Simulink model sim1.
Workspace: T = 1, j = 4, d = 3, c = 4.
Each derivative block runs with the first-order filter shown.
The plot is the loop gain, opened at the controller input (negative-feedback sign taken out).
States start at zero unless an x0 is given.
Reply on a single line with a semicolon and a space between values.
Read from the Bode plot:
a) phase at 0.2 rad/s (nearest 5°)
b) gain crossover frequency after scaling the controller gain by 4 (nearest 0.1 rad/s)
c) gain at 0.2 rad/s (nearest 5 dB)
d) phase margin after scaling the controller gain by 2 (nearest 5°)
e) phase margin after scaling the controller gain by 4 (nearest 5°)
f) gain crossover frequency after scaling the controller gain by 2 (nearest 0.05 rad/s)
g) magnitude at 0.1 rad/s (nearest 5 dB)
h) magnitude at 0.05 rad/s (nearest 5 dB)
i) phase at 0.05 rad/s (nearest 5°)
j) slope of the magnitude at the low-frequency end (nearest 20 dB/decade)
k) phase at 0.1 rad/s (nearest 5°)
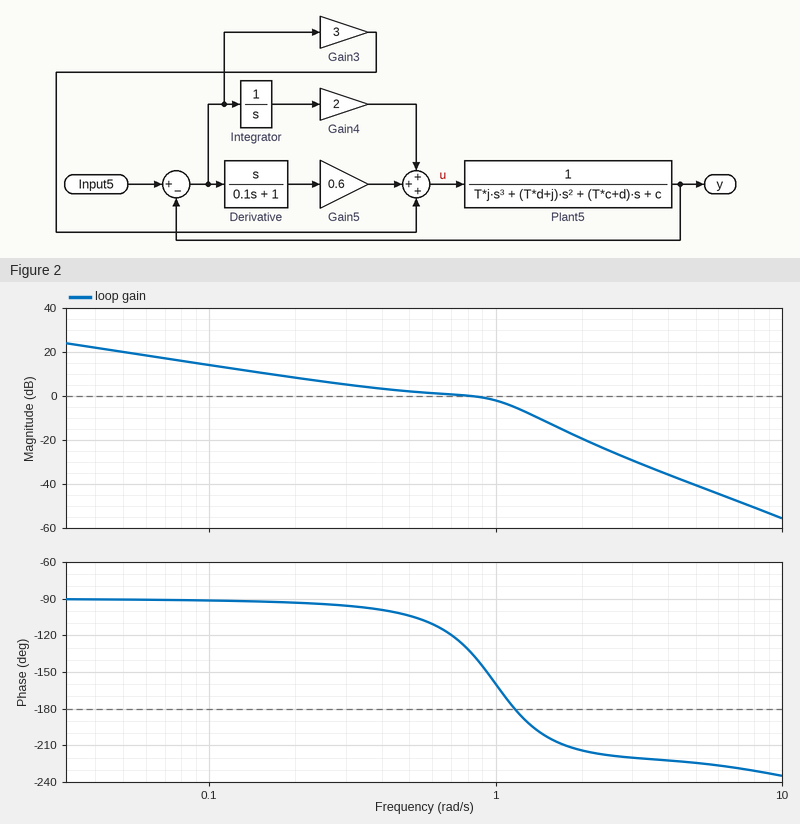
-95°; 1.5 rad/s; 10 dB; -5°; -25°; 1.20 rad/s; 15 dB; 20 dB; -90°; -20 dB/decade; -90°
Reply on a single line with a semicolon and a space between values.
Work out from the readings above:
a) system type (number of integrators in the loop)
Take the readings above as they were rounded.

1
